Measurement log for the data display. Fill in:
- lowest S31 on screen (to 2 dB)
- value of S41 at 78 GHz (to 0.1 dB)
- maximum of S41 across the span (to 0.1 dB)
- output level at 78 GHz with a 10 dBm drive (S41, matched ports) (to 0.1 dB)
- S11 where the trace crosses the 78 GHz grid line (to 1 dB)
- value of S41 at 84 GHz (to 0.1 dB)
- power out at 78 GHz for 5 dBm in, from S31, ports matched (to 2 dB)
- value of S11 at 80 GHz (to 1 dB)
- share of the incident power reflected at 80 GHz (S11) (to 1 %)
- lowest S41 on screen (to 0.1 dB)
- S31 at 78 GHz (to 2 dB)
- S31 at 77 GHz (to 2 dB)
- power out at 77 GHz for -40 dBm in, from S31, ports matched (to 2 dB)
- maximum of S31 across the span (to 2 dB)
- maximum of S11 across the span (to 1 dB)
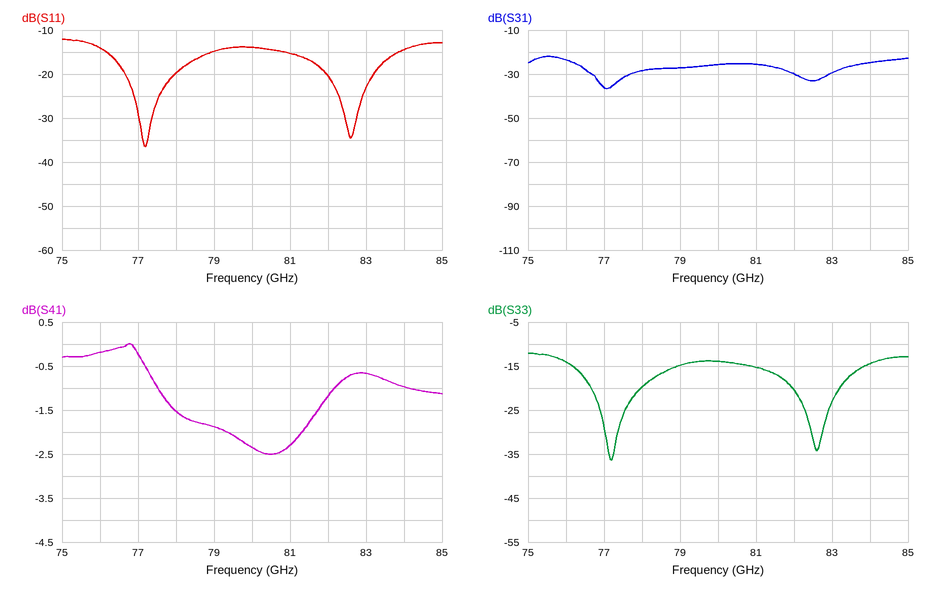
-36 dB
-1.5 dB
0.0 dB
8.5 dBm
-20 dB
-1.0 dB
-24 dBm
-14 dB
4 %
-2.5 dB
-28 dB
-36 dB
-76 dBm
-22 dB
-12 dB
